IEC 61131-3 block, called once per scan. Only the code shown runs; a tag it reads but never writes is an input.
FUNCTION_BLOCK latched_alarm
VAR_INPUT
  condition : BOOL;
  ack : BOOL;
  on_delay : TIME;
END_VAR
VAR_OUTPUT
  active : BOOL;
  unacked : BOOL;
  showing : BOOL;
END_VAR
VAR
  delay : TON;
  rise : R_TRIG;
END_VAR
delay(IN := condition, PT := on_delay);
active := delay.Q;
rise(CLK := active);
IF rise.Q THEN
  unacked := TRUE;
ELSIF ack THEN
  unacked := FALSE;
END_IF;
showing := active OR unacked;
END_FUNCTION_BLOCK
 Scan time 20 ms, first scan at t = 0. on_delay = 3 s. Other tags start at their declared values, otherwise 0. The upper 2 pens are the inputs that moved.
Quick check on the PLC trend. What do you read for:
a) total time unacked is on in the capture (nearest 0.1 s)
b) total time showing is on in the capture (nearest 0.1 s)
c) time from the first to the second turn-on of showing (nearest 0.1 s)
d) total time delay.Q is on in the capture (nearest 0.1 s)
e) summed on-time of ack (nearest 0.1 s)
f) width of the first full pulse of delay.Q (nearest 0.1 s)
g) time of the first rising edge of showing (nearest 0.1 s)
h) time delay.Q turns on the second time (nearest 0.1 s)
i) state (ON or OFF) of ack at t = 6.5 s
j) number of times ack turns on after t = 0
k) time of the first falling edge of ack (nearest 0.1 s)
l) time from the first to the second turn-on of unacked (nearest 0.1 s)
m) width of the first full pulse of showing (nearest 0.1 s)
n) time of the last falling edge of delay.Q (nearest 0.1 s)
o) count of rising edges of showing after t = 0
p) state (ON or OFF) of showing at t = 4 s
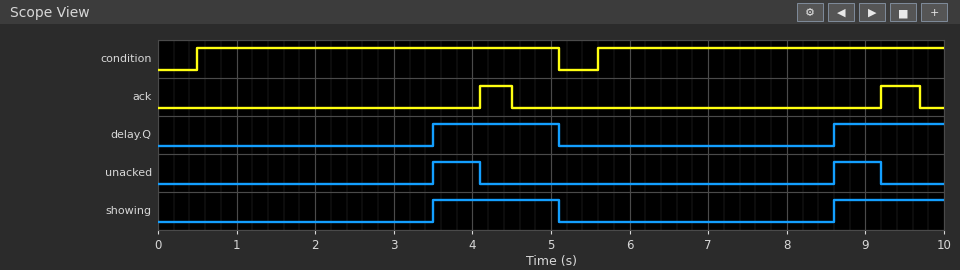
1.2 s
3.0 s
5.1 s
3.0 s
0.9 s
1.6 s
3.5 s
8.6 s
OFF
2
4.5 s
5.1 s
1.6 s
5.1 s
2
ON
